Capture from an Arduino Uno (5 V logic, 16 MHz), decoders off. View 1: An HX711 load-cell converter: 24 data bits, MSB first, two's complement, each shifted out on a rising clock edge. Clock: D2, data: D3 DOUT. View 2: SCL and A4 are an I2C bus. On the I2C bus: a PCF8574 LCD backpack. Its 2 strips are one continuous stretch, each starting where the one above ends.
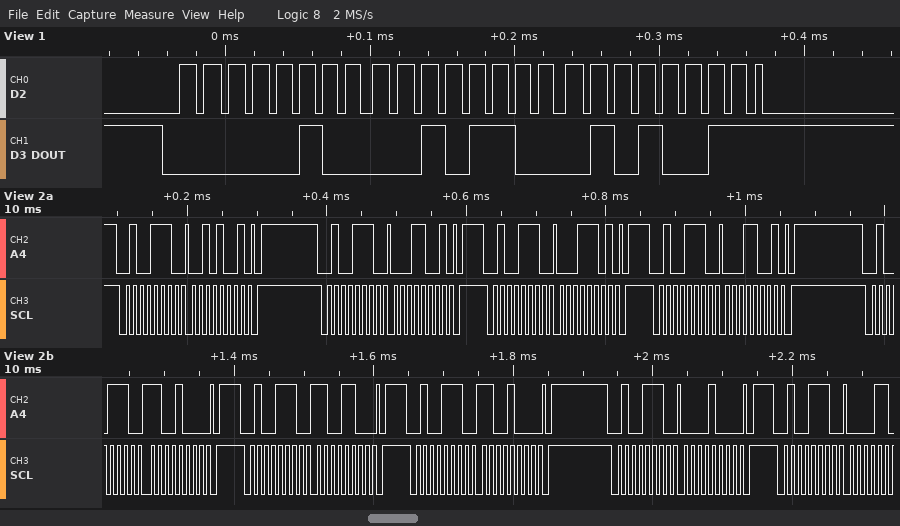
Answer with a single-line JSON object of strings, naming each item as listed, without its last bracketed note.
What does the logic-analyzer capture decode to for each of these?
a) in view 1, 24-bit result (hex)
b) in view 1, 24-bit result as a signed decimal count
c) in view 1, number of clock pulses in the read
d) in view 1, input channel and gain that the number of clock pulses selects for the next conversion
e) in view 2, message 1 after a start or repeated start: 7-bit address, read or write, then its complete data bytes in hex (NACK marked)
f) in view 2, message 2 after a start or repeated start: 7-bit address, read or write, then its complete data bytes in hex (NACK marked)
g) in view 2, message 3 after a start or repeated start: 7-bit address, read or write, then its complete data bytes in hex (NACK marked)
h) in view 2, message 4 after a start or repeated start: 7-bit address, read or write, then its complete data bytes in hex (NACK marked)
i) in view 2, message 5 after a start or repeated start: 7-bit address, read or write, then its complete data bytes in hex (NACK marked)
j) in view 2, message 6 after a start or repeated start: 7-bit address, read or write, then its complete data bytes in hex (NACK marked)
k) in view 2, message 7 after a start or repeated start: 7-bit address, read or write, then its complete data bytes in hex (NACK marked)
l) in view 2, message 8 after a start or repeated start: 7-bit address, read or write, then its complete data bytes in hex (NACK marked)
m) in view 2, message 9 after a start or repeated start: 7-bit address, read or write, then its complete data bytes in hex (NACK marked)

{"in view 1, 24-bit result": "0x042C53", "in view 1, 24-bit result as a signed decimal count": "273491", "in view 1, number of clock pulses in the read": "25", "in view 1, input channel and gain that the number of clock pulses selects for the next conversion": "channel A, gain 128", "in view 2, message 1 after a start or repeated start: 7-bit address, read or write, then its complete data bytes in hex": "0x27 write: 29", "in view 2, message 2 after a start or repeated start: 7-bit address, read or write, then its complete data bytes in hex": "0x27 write: 19", "in view 2, message 3 after a start or repeated start: 7-bit address, read or write, then its complete data bytes in hex": "0x27 write: 1D", "in view 2, message 4 after a start or repeated start: 7-bit address, read or write, then its complete data bytes in hex": "0x27 write: 19", "in view 2, message 5 after a start or repeated start: 7-bit address, read or write, then its complete data bytes in hex": "0x27 write: C8", "in view 2, message 6 after a start or repeated start: 7-bit address, read or write, then its complete data bytes in hex": "0x27 write: CC", "in view 2, message 7 after a start or repeated start: 7-bit address, read or write, then its complete data bytes in hex": "0x27 write: C8", "in view 2, message 8 after a start or repeated start: 7-bit address, read or write, then its complete data bytes in hex": "0x27 write: 08", "in view 2, message 9 after a start or repeated start: 7-bit address, read or write, then its complete data bytes in hex": "0x27 write"}
